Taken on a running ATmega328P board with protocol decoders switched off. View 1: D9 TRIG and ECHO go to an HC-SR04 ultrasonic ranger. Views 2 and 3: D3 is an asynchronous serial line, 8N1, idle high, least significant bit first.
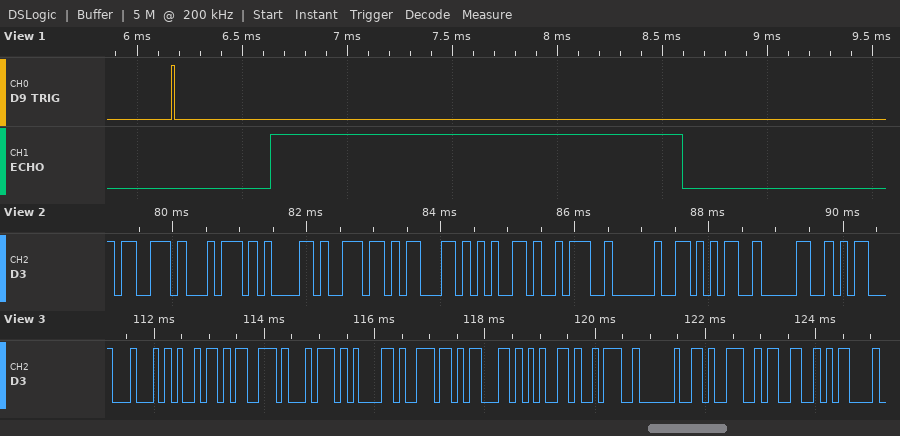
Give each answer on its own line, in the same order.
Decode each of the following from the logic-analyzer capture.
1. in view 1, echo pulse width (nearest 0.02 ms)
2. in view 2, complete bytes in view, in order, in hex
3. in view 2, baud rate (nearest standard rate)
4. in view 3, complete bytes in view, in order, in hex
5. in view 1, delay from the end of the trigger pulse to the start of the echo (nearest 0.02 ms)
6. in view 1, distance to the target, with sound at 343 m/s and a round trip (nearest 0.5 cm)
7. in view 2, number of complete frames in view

1.96 ms
73 74 61 6E 63 65 3A 20 35 30
9600 baud
0x44 0x69 0x73 0x74 0x61 0x6E 0x63 0x65 0x3A 0x20 0x39 0x33 0x0D
0.46 ms
33.5 cm
10
